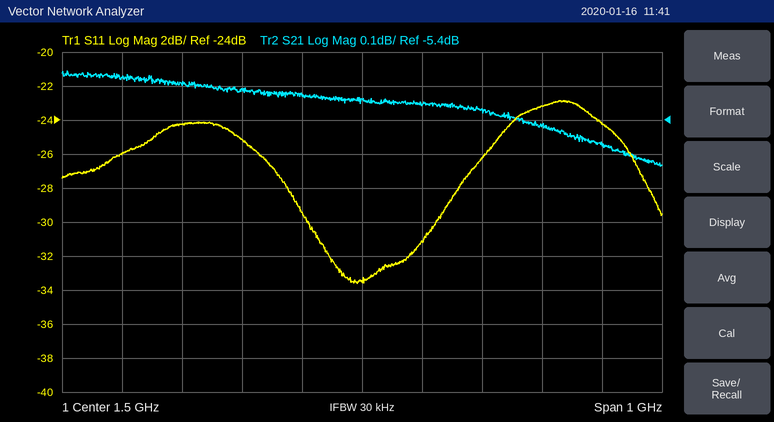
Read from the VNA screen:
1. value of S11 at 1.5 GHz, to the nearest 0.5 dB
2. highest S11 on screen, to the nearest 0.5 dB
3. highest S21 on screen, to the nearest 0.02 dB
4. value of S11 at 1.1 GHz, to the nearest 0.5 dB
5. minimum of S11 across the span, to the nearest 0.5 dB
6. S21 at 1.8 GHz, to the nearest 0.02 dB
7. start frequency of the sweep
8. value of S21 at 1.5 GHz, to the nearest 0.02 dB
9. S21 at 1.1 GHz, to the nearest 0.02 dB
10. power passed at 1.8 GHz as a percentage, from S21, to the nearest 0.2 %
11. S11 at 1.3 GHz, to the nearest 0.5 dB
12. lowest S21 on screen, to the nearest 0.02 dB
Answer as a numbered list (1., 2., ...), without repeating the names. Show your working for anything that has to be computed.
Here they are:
1. -33.5 dB
2. -23.0 dB
3. -5.26 dB
4. -26.0 dB
5. -33.5 dB
6. -5.42 dB
7. 1 GHz
8. -5.34 dB
9. -5.28 dB
10. 10^(-5.42/10) ≈ 28.7 %, so 28.8 % to the nearest 0.2 %
11. -25.0 dB
12. -5.54 dB
